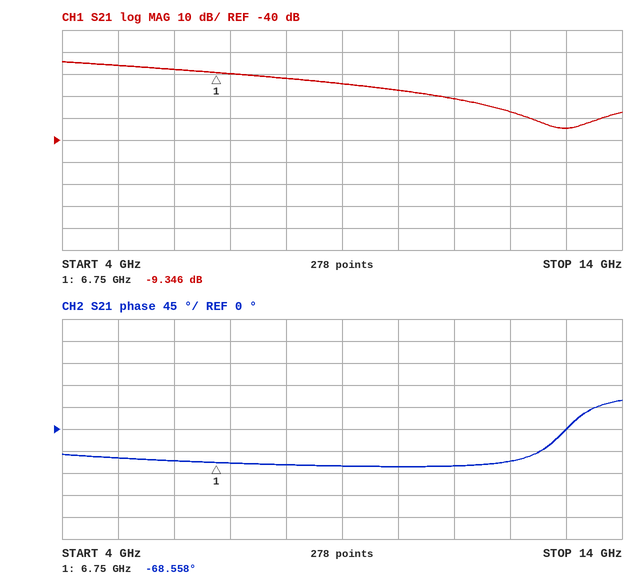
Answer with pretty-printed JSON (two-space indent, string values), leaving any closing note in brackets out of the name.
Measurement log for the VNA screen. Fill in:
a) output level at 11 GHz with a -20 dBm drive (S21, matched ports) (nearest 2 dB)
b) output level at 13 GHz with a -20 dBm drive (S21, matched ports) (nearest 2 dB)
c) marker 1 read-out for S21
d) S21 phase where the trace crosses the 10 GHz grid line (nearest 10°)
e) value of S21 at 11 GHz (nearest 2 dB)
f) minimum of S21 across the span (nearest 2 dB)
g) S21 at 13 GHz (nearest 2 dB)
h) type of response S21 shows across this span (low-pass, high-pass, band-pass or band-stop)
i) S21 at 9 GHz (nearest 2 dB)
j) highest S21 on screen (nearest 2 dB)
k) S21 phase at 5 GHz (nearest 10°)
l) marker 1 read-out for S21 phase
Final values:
{
  "output level at 11 GHz with a -20 dBm drive (S21, matched ports)": "-42 dBm",
  "output level at 13 GHz with a -20 dBm drive (S21, matched ports)": "-54 dBm",
  "marker 1 read-out for S21": "-9.346 dB",
  "S21 phase where the trace crosses the 10 GHz grid line": "-80°",
  "value of S21 at 11 GHz": "-22 dB",
  "minimum of S21 across the span": "-34 dB",
  "S21 at 13 GHz": "-34 dB",
  "type of response S21 shows across this span": "low-pass",
  "S21 at 9 GHz": "-14 dB",
  "highest S21 on screen": "-4 dB",
  "S21 phase at 5 GHz": "-60°",
  "marker 1 read-out for S21 phase": "-68.558°"
}
